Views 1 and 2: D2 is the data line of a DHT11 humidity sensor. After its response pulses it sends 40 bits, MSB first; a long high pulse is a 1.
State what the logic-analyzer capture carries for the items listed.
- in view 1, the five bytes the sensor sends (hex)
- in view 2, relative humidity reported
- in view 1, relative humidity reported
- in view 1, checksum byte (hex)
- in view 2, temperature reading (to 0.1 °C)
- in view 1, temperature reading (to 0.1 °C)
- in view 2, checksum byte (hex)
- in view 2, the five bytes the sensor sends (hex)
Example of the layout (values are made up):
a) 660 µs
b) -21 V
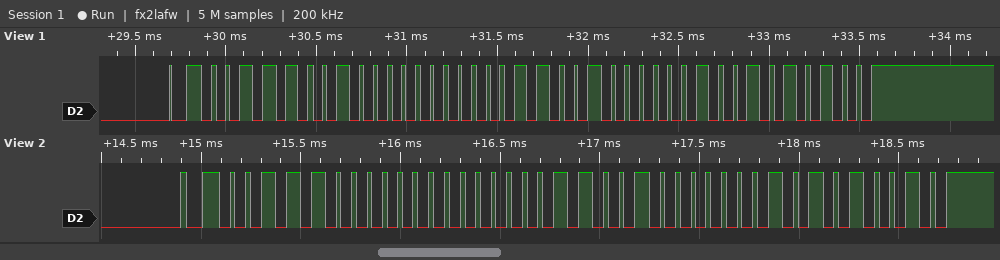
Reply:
a) 39 00 19 02 54
b) 56 %
c) 57 %
d) 0x54
e) 25.1 °C
f) 25.2 °C
g) 0x52
h) 38 00 19 01 52
